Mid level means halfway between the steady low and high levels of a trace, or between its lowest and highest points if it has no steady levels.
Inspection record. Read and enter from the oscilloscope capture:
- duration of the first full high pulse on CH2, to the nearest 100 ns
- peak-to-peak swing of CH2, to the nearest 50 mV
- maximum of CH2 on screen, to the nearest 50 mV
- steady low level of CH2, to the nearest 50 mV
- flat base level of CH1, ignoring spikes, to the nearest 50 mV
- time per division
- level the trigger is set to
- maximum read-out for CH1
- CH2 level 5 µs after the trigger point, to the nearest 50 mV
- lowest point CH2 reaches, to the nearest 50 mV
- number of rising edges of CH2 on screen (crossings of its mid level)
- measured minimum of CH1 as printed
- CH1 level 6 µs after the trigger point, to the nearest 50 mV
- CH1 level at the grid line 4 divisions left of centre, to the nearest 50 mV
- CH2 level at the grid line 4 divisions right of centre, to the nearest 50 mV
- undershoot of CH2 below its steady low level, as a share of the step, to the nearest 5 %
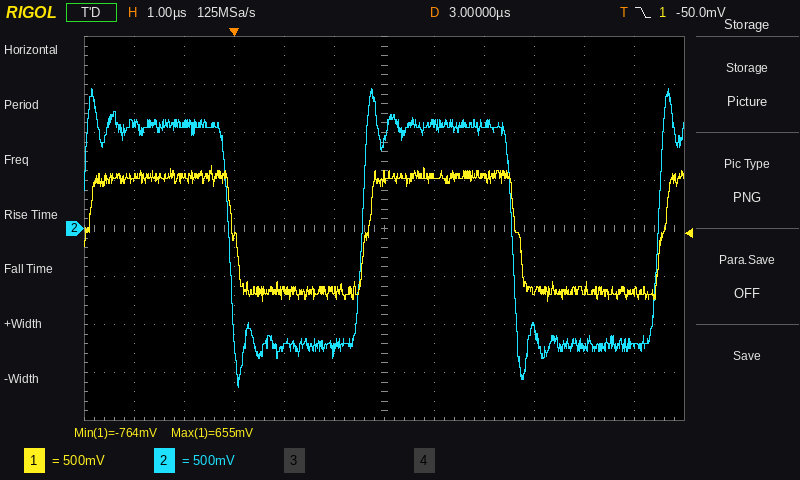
3.0 µs
3.10 V
1.45 V
-1.20 V
-650 mV
1 µs
-50.0 mV
655 mV
1.10 V
-1.65 V
2
-764 mV
-650 mV
550 mV
-1.25 V
20 %
